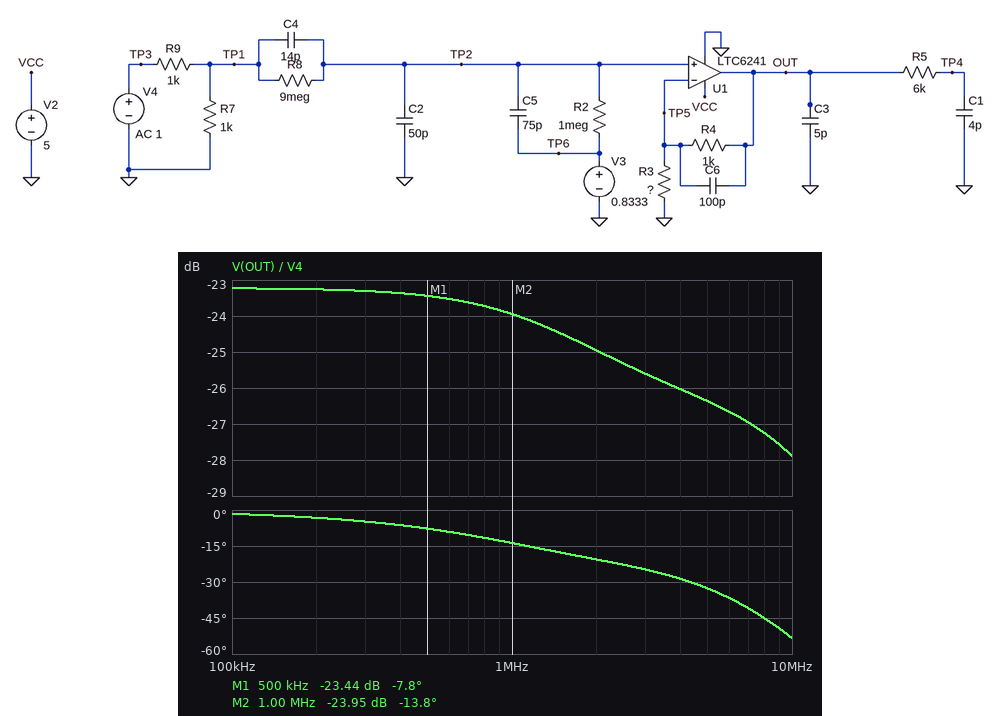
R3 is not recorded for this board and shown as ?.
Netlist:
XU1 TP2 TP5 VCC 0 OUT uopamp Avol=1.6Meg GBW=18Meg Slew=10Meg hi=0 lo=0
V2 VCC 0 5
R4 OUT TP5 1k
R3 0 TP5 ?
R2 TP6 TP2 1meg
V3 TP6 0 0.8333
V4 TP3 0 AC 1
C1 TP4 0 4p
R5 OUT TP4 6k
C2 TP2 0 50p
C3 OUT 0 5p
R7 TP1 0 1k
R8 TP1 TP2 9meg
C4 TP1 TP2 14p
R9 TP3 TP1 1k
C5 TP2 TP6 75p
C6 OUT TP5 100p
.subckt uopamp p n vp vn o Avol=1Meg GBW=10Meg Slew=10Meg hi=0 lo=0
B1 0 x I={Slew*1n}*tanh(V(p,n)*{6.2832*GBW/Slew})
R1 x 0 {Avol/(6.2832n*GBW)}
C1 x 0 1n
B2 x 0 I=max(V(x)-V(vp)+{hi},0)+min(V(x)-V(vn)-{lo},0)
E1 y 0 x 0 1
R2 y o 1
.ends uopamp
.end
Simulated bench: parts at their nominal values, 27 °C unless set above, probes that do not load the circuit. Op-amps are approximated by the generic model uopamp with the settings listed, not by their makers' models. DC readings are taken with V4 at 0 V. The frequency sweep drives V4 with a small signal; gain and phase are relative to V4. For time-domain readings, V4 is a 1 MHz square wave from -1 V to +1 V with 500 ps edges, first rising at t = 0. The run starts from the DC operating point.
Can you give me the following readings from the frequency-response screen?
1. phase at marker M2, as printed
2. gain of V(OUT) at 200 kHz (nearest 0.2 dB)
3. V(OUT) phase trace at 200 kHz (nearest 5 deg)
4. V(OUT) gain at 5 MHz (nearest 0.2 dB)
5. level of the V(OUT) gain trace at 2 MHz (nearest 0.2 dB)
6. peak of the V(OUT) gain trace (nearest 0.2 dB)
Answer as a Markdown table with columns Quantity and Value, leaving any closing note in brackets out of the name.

| Quantity | Value |
|---|---|
| phase at marker M2, as printed | -13.8 deg |
| gain of V(OUT) at 200 kHz | -23.2 dB |
| V(OUT) phase trace at 200 kHz | -5 deg |
| V(OUT) gain at 5 MHz | -26.4 dB |
| level of the V(OUT) gain trace at 2 MHz | -25.0 dB |
| peak of the V(OUT) gain trace | -23.2 dB |
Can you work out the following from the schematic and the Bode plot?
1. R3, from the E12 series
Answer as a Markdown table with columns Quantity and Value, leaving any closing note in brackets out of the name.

| Quantity | Value |
|---|---|
| R3, from the E12 series | 2.7 kΩ |
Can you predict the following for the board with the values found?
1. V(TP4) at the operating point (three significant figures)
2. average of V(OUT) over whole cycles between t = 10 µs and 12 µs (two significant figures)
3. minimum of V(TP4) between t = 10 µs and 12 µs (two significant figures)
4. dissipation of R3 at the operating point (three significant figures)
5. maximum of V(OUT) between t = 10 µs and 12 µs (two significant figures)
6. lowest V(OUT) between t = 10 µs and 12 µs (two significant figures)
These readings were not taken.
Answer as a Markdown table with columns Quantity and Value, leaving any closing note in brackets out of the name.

| Quantity | Value |
|---|---|
| V(TP4) at the operating point | 1.03 V |
| average of V(OUT) over whole cycles between t = 10 µs and 12 µs | 1.0 V |
| minimum of V(TP4) between t = 10 µs and 12 µs | 960 mV |
| dissipation of R3 at the operating point | 208 µW |
| maximum of V(OUT) between t = 10 µs and 12 µs | 1.1 V |
| lowest V(OUT) between t = 10 µs and 12 µs | 960 mV |
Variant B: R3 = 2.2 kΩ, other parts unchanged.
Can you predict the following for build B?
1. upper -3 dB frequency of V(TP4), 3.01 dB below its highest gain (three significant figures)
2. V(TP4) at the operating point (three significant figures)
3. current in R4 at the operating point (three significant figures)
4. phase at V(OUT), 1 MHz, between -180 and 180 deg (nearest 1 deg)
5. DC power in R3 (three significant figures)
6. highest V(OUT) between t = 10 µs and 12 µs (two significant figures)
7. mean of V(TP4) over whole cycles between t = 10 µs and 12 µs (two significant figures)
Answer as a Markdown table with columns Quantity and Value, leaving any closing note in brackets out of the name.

| Quantity | Value |
|---|---|
| upper -3 dB frequency of V(TP4), 3.01 dB below its highest gain | 2.50 MHz |
| V(TP4) at the operating point | 1.09 V |
| current in R4 at the operating point | 341 µA |
| phase at V(OUT), 1 MHz, between -180 and 180 deg | -15 deg |
| DC power in R3 | 256 µW |
| highest V(OUT) between t = 10 µs and 12 µs | 1.2 V |
| mean of V(TP4) over whole cycles between t = 10 µs and 12 µs | 1.1 V |
